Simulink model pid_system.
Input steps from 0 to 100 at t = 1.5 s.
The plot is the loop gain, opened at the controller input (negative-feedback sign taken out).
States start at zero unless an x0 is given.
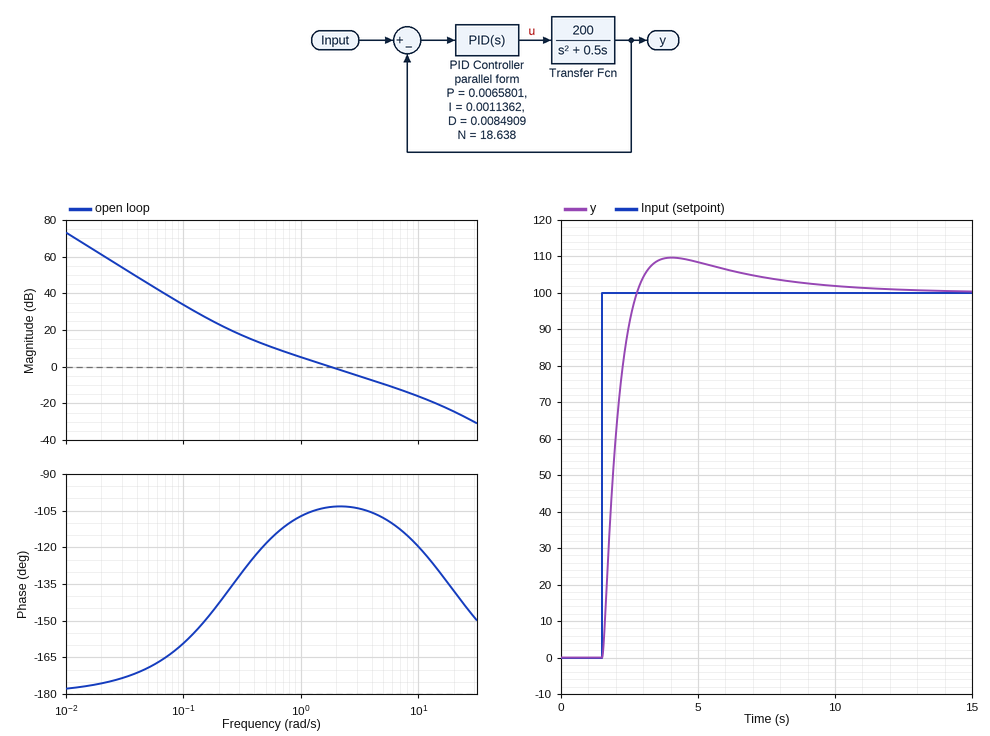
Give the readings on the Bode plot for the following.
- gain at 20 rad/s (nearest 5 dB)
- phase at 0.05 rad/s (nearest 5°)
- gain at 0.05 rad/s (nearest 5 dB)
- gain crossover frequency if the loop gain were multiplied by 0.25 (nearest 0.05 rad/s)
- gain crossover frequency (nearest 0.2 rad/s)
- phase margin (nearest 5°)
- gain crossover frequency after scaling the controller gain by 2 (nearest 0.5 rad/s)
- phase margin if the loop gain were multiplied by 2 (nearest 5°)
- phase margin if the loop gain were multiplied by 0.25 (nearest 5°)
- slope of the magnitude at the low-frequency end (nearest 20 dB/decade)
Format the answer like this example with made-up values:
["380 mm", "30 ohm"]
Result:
["-25 dB", "-170°", "45 dB", "0.50 rad/s", "1.8 rad/s", "75°", "3.5 rad/s", "75°", "60°", "-40 dB/decade"]
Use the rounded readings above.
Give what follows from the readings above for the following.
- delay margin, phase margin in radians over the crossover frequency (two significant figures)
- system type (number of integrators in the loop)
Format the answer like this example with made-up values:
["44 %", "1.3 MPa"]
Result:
["0.73 s", "2"]
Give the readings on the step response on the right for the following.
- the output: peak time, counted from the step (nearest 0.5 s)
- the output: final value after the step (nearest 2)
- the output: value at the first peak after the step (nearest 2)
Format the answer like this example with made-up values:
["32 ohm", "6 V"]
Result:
["2.5 s", "100", "110"]
